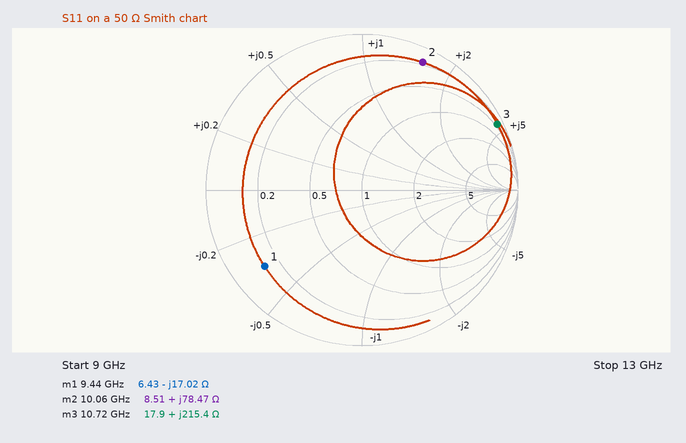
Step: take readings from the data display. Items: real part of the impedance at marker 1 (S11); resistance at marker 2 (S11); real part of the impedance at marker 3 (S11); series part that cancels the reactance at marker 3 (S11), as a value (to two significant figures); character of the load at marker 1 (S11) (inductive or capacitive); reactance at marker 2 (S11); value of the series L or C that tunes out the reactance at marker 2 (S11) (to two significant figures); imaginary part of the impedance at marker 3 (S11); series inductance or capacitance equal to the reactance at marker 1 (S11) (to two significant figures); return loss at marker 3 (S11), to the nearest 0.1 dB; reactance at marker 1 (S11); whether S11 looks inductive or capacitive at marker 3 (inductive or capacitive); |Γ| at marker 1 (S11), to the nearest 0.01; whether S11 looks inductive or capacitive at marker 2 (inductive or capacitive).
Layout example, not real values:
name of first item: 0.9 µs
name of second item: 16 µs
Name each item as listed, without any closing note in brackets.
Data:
real part of the impedance at marker 1: 6.43 Ω
resistance at marker 2: 8.51 Ω
real part of the impedance at marker 3: 17.9 Ω
series part that cancels the reactance at marker 3 (S11), as a value: 69 fF
character of the load at marker 1 (S11): capacitive
reactance at marker 2: +78.47 Ω
value of the series L or C that tunes out the reactance at marker 2 (S11): 200 fF
imaginary part of the impedance at marker 3: +215.4 Ω
series inductance or capacitance equal to the reactance at marker 1 (S11): 990 fF
return loss at marker 3 (S11), to the nearest 0.1 dB: 0.3 dB
reactance at marker 1: -17.02 Ω
whether S11 looks inductive or capacitive at marker 3: inductive
|Γ| at marker 1 (S11), to the nearest 0.01: 0.79
whether S11 looks inductive or capacitive at marker 2: inductive
